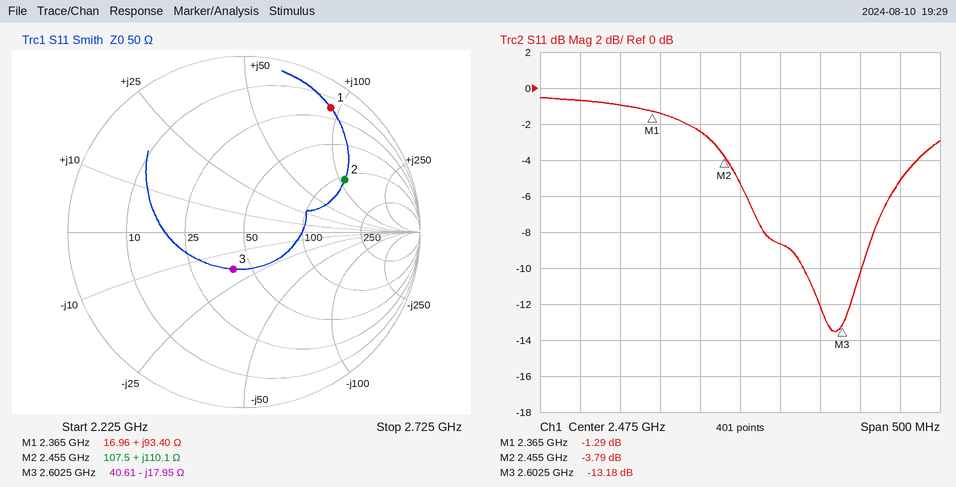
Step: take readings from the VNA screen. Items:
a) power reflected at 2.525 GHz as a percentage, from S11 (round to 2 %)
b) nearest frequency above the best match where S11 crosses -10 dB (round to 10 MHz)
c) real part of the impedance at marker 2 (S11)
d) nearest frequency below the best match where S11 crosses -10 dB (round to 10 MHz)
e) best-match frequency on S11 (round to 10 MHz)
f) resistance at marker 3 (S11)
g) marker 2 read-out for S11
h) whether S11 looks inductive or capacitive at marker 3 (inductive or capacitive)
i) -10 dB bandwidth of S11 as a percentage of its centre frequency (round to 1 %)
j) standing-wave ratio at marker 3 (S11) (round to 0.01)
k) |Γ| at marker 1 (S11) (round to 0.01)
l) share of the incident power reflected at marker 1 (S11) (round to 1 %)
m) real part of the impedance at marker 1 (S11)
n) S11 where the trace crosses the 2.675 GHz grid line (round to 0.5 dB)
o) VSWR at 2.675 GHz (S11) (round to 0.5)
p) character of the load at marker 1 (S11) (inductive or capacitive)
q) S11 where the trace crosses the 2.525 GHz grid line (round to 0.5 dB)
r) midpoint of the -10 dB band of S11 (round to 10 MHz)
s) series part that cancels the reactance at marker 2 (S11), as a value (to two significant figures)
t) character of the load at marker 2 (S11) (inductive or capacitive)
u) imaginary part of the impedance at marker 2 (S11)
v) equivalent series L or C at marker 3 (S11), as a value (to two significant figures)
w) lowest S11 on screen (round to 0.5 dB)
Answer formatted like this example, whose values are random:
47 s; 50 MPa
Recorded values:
14 %; 2.63 GHz; 107.5 Ω; 2.55 GHz; 2.59 GHz; 40.61 Ω; -3.79 dB; capacitive; 3 %; 1.56; 0.86; 74 %; 16.96 Ω; -5.0 dB; 3.5; inductive; -8.5 dB; 2.59 GHz; 590 fF; inductive; +110.1 Ω; 3.4 pF; -13.5 dB
